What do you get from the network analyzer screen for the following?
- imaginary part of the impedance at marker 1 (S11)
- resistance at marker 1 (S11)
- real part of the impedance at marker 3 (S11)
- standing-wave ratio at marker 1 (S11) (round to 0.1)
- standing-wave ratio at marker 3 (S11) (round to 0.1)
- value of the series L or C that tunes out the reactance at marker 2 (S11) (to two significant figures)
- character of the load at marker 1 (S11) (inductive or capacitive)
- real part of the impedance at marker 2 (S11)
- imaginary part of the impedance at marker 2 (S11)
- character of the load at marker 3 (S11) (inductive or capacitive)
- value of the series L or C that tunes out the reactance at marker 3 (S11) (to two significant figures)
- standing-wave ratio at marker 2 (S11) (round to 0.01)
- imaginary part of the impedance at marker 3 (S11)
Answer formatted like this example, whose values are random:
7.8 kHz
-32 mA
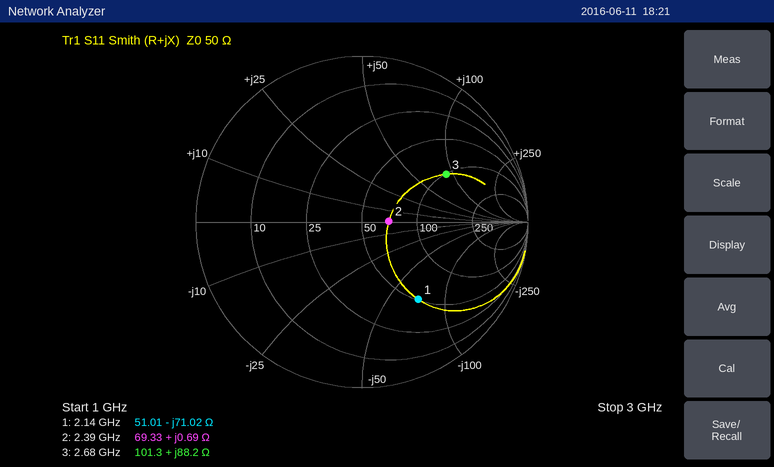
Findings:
-71.02 Ω
51.01 Ω
101.3 Ω
3.7
3.8
97 pF
capacitive
69.33 Ω
+0.69 Ω
inductive
670 fF
1.39
+88.2 Ω
